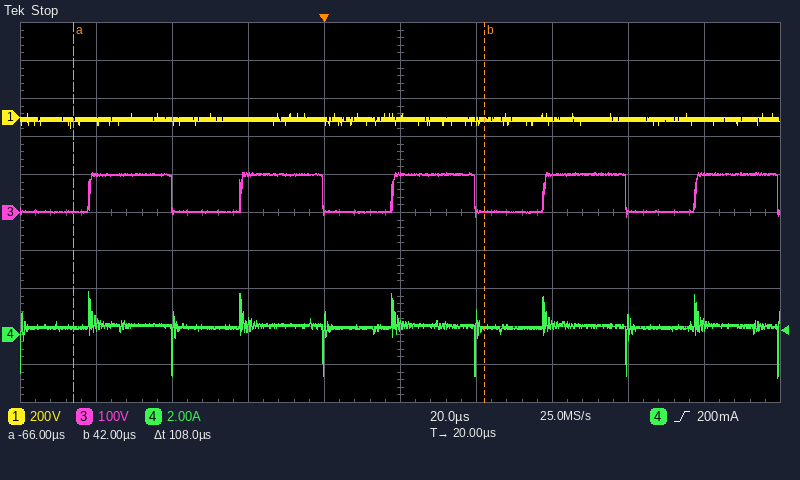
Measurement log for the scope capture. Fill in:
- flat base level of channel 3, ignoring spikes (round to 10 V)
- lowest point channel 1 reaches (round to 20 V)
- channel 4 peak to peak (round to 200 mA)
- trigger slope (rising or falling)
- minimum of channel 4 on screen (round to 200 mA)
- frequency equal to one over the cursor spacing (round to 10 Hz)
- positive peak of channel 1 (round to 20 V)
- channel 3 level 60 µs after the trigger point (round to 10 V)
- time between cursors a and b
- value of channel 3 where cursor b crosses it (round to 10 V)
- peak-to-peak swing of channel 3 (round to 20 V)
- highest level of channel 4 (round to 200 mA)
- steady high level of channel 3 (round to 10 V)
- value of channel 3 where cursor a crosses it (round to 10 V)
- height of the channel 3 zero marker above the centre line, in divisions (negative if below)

0 V
-60 V
4.6 A
rising
-2.4 A
9.26 kHz
20 V
100 V
108 µs
0 V
120 V
2.2 A
100 V
0 V
0.0 div
